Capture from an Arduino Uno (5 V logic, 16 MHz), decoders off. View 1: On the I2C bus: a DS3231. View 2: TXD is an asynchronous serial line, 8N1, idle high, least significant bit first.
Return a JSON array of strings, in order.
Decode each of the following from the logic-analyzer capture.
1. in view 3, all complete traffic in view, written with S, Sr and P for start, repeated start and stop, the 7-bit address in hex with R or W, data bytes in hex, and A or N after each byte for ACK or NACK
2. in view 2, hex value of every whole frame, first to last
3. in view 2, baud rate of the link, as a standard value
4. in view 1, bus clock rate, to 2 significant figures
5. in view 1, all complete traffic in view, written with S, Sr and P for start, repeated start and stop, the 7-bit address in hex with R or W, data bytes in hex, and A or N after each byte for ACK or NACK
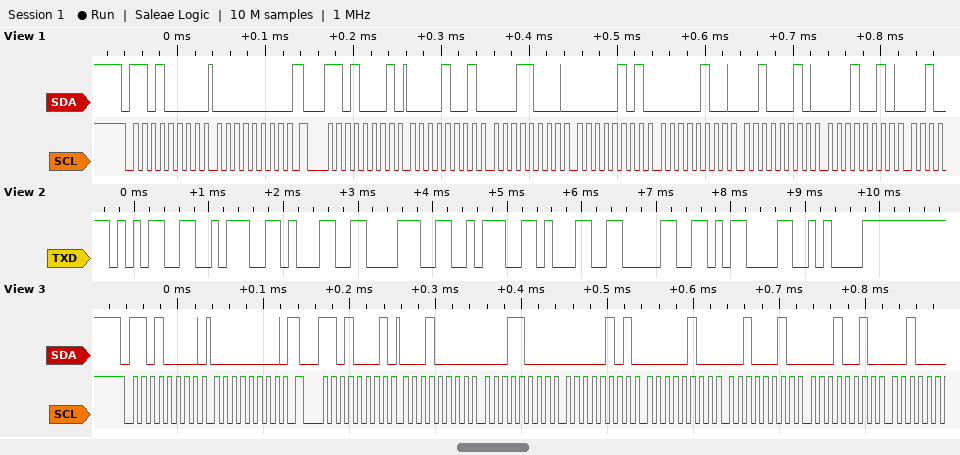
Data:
["S 68W A 00 A Sr 68R A 10 A 18 A 05 A 04 A 22 A 12 A", "35 3A 31 38 3A 31 30 0D 0A", "9600 baud", "100 kHz", "S 68W A 00 A Sr 68R A 09 A 18 A 05 A 04 A 22 A 12 A"]
